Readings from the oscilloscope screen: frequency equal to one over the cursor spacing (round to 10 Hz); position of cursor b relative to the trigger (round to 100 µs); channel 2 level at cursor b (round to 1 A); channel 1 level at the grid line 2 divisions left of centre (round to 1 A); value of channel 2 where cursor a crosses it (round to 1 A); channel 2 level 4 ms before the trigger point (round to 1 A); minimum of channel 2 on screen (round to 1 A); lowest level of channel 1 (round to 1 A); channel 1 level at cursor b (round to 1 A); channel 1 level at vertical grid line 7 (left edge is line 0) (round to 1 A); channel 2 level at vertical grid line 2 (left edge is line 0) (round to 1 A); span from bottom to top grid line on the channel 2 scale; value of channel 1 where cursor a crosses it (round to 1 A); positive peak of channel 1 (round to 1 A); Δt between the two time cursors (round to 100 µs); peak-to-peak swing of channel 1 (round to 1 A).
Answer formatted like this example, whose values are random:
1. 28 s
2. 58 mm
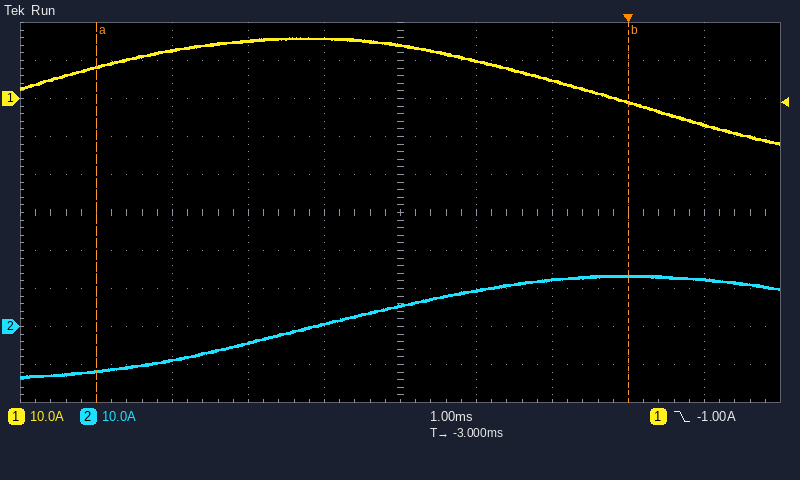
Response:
1. 140 Hz
2. 0.0 ms
3. 13 A
4. 15 A
5. -12 A
6. 1 A
7. -13 A
8. -12 A
9. -1 A
10. 5 A
11. -9 A
12. 100 A
13. 8 A
14. 16 A
15. 7.0 ms
16. 28 A
